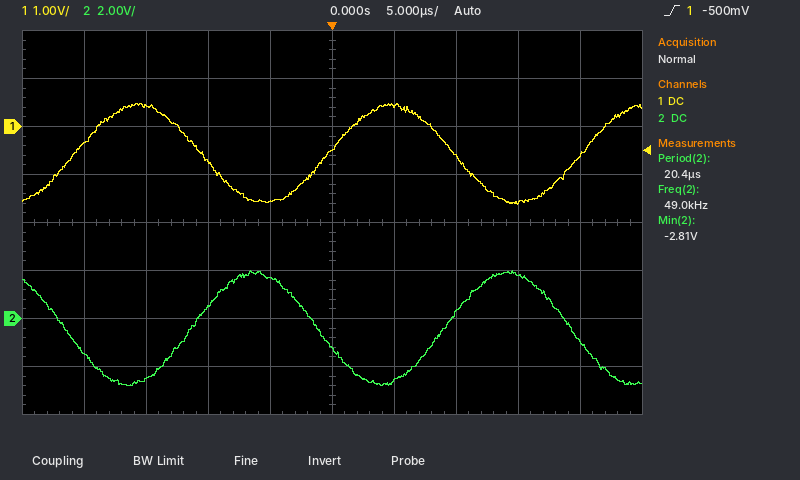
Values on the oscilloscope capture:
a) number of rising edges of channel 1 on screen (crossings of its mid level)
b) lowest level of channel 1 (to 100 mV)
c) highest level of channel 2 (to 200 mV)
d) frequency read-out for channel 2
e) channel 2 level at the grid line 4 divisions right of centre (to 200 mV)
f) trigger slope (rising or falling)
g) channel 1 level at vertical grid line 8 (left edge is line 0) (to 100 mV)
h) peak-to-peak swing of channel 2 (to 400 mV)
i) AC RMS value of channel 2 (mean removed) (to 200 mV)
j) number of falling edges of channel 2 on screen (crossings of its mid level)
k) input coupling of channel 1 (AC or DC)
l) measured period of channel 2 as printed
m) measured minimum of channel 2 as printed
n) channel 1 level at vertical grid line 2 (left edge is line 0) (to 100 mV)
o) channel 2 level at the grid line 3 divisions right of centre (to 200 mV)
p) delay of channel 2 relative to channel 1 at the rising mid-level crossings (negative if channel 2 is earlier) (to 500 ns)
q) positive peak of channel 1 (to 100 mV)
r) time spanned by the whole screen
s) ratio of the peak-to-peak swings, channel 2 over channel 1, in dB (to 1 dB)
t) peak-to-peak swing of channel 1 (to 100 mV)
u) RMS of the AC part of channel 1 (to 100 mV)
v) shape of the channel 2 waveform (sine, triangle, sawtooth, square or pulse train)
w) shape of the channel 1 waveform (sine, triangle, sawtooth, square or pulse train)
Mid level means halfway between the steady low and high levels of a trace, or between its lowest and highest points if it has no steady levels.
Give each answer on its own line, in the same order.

3
-1.6 V
2.0 V
49.0 kHz
-1.0 V
rising
-1.6 V
4.8 V
1.6 V
3
DC
20.4 µs
-2.81 V
400 mV
1.8 V
+9.5 µs
500 mV
50 µs
7 dB
2.1 V
700 mV
sine
sine
